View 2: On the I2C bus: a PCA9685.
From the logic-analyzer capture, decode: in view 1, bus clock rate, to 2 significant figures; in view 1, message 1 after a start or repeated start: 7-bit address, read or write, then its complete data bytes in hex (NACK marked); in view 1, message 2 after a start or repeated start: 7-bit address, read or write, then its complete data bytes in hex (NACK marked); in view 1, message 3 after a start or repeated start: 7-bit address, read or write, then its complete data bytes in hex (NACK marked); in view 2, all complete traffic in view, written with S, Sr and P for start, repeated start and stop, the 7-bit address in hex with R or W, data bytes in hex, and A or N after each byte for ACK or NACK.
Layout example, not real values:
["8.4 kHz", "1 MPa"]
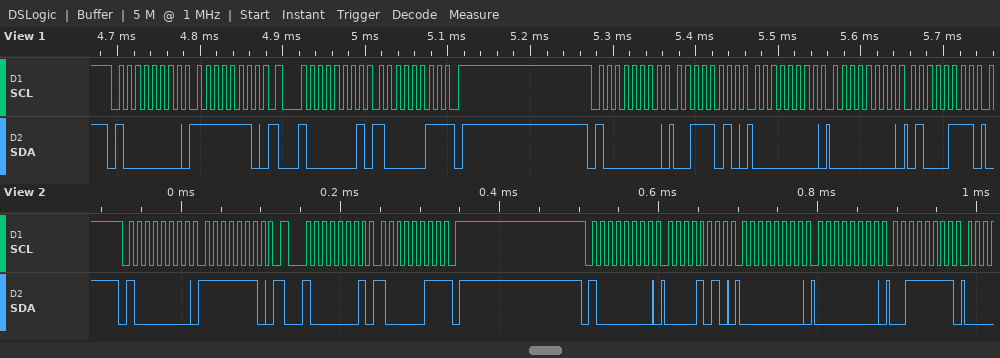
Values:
["100 kHz", "0x40 write: FE", "0x40 read: 83 NACK", "0x40 write: 3A 00 00 47", "S 40W A FE A Sr 40R A 83 N P S 40W A 0A A 00 A 00 A 3F A"]
